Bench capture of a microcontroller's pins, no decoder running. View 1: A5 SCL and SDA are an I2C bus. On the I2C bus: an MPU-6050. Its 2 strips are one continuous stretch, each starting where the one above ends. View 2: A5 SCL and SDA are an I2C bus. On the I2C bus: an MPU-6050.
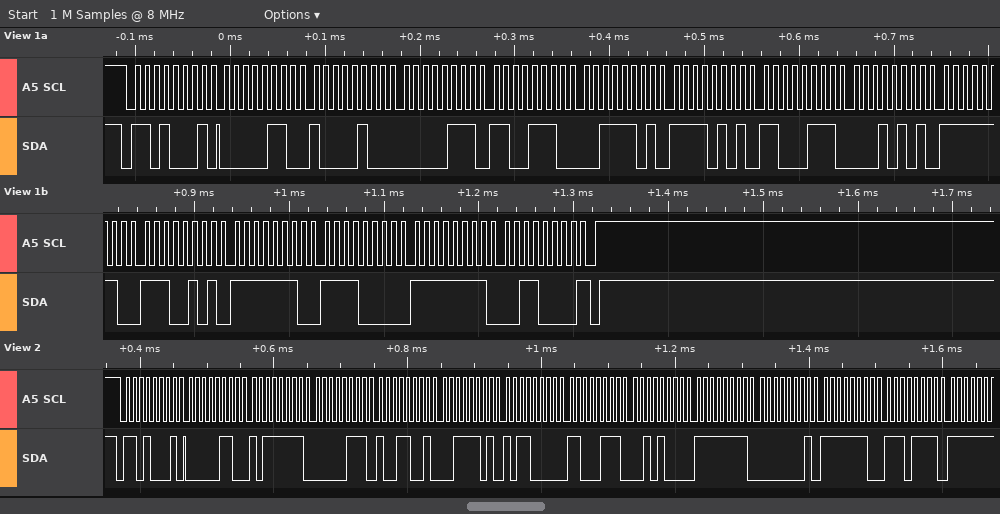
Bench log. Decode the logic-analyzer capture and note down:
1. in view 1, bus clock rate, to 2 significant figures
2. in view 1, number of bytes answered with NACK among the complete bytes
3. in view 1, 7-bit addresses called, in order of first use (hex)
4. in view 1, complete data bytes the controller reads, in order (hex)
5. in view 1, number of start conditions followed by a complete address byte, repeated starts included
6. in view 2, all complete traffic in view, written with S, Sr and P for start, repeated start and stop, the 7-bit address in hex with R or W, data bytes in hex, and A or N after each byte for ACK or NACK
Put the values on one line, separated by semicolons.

100 kHz; 1; 0x68; 06 84 07 CE 3D F5 C7 15 FE E5 FE F0 FF 30; 1; S 68R A 06 A BF A 07 A 99 A 3D A B0 A C7 A 28 A FF A 01 A FE A EF A
